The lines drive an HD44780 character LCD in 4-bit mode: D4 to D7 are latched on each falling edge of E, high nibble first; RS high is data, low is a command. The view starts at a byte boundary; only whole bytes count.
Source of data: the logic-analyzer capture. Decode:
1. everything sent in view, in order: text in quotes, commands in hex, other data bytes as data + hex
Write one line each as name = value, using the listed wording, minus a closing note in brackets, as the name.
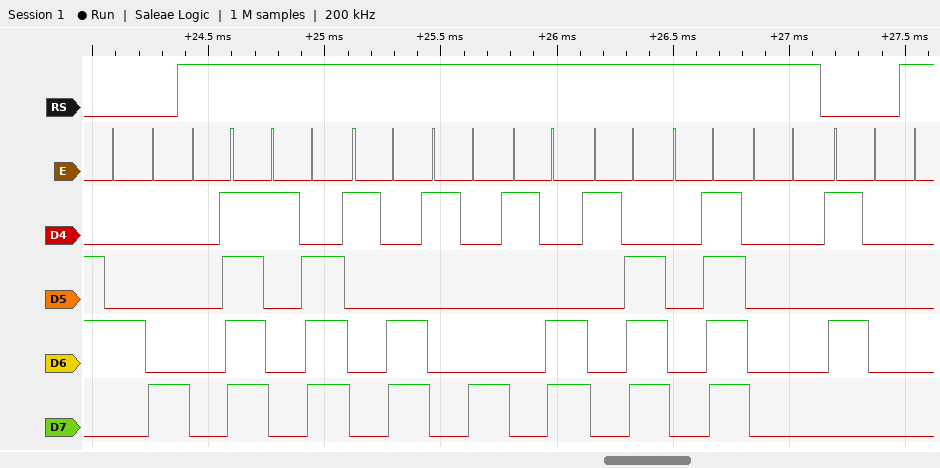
everything sent in view, in order: text in quotes, commands in hex, other data bytes as data + hex = 0x48 data 0F 1E 1C 18 1C 1E 0F 00 0x50
